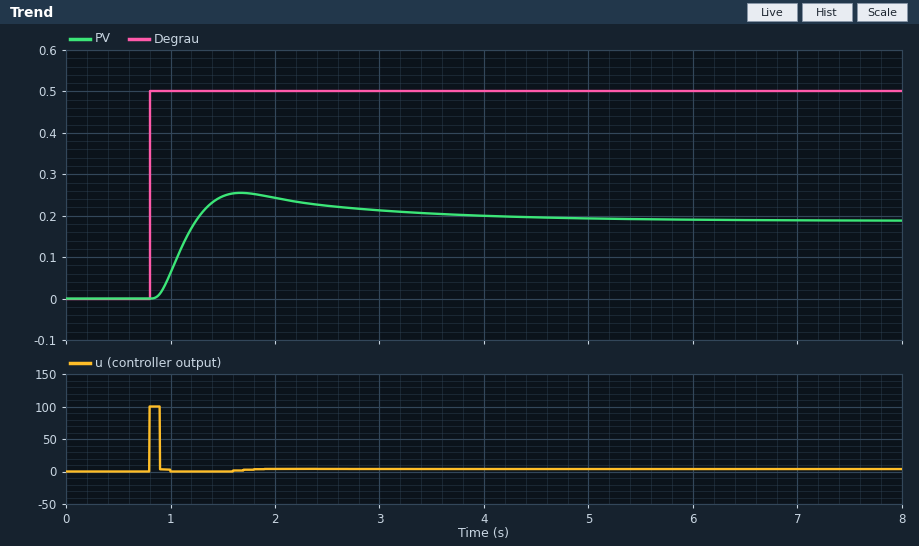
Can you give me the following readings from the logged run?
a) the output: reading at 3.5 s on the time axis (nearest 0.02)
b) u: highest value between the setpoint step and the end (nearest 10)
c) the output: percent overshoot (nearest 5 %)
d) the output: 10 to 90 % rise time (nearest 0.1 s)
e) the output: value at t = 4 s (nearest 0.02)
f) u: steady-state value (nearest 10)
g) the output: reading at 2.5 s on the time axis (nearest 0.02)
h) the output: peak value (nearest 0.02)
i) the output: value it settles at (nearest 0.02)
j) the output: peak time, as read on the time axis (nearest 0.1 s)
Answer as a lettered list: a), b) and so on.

a) 0.20
b) 100
c) 35 %
d) 0.3 s
e) 0.20
f) 0
g) 0.22
h) 0.26
i) 0.18
j) 1.7 s
